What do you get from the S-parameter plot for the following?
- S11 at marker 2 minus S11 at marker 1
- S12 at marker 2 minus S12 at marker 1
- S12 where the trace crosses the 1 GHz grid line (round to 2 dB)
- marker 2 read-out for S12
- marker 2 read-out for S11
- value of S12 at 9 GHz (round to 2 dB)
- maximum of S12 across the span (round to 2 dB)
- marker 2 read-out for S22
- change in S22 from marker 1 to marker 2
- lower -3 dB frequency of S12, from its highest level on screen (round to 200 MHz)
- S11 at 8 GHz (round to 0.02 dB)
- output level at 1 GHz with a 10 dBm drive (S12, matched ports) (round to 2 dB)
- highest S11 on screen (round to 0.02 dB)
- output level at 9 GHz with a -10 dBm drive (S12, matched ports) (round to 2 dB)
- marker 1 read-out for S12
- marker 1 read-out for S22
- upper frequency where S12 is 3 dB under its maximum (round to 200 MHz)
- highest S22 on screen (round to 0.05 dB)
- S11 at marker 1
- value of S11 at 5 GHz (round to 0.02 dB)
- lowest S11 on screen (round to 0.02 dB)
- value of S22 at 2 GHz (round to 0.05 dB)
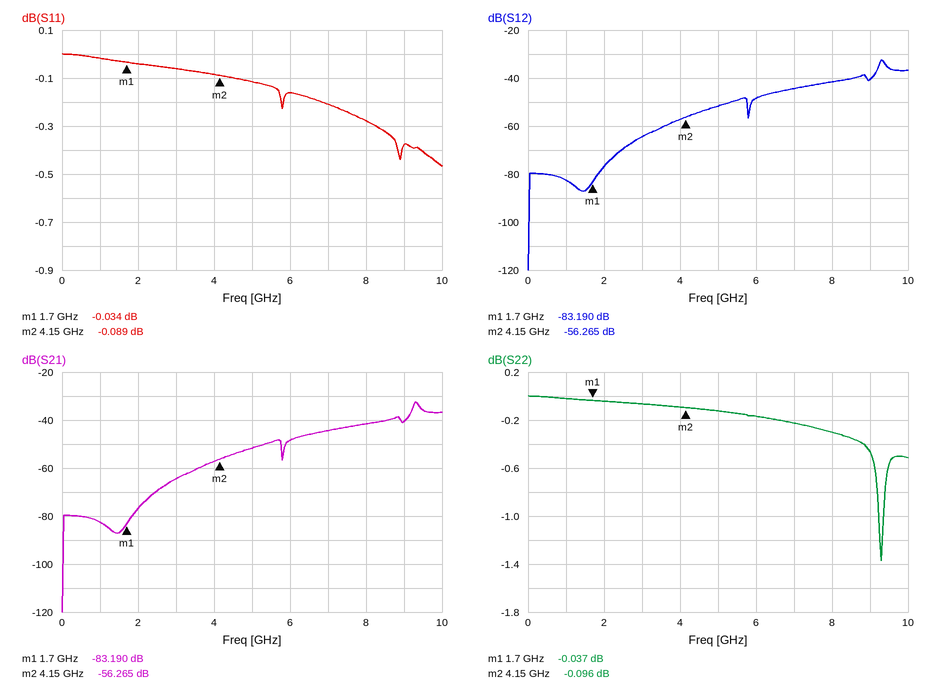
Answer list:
-0.055 dB
26.925 dB
-82 dB
-56.265 dB
-0.089 dB
-40 dB
-32 dB
-0.096 dB
-0.059 dB
9.2 GHz
-0.28 dB
-72 dBm
0.00 dB
-50 dBm
-83.190 dB
-0.037 dB
9.4 GHz
0.00 dB
-0.034 dB
-0.12 dB
-0.46 dB
-0.05 dB
